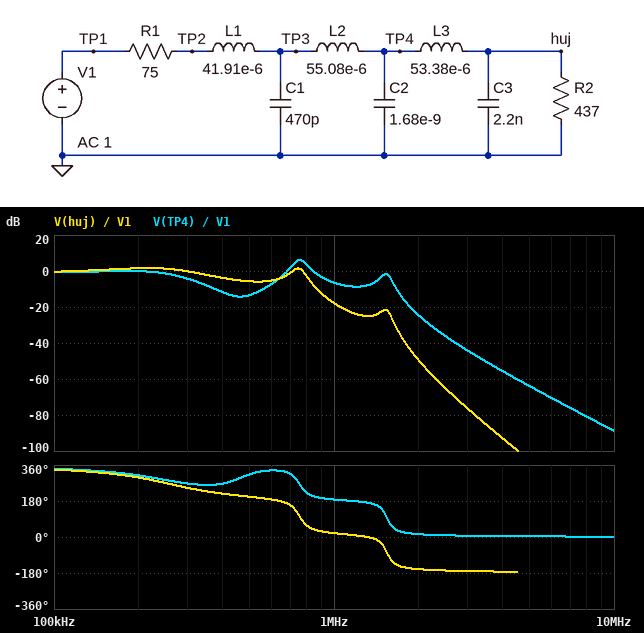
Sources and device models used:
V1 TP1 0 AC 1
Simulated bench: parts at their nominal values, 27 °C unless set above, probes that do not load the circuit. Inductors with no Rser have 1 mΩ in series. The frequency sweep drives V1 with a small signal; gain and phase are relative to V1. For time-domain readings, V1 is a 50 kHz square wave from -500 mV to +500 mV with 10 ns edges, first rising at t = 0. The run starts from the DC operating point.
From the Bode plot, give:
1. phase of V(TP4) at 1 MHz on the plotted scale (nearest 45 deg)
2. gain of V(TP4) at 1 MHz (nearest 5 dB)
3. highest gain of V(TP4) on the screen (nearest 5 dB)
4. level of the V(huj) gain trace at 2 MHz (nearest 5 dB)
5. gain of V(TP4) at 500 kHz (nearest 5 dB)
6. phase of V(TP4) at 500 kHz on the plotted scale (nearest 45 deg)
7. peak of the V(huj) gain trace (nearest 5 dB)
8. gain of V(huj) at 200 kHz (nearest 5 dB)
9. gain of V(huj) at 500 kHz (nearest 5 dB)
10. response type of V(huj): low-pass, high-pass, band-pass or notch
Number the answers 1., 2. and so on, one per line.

1. 180 deg
2. -5 dB
3. 5 dB
4. -50 dB
5. -15 dB
6. 315 deg
7. 0 dB
8. 0 dB
9. -5 dB
10. low-pass
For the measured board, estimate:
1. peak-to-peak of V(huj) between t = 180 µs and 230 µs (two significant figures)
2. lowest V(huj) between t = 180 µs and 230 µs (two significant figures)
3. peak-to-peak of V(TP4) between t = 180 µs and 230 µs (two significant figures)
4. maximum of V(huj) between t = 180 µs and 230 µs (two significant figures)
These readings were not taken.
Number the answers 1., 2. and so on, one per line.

1. 1.3 V
2. -670 mV
3. 1.5 V
4. 670 mV
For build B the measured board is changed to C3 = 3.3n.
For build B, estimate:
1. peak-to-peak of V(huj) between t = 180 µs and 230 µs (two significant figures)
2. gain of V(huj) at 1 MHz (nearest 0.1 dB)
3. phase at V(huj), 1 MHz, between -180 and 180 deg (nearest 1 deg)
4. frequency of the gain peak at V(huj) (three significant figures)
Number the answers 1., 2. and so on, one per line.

1. 1.4 V
2. -22.4 dB
3. 13 deg
4. 186 kHz
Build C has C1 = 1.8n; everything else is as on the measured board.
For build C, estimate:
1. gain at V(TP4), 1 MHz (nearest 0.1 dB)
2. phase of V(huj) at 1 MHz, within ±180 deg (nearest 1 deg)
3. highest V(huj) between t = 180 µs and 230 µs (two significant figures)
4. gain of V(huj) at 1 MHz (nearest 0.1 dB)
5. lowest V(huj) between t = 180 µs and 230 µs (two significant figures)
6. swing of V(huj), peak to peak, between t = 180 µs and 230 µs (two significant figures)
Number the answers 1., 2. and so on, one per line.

1. -0.8 dB
2. -128 deg
3. 700 mV
4. -12.2 dB
5. -700 mV
6. 1.4 V
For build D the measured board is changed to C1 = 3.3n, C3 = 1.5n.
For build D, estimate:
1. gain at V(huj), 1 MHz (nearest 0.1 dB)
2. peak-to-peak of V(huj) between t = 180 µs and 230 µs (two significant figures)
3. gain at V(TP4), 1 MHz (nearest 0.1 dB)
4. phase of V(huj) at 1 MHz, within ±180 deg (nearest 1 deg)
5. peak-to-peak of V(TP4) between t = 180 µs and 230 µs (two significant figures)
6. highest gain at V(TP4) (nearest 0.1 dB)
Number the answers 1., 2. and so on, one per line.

1. -19.2 dB
2. 1.5 V
3. -12.0 dB
4. -131 deg
5. 1.2 V
6. 1.8 dB
